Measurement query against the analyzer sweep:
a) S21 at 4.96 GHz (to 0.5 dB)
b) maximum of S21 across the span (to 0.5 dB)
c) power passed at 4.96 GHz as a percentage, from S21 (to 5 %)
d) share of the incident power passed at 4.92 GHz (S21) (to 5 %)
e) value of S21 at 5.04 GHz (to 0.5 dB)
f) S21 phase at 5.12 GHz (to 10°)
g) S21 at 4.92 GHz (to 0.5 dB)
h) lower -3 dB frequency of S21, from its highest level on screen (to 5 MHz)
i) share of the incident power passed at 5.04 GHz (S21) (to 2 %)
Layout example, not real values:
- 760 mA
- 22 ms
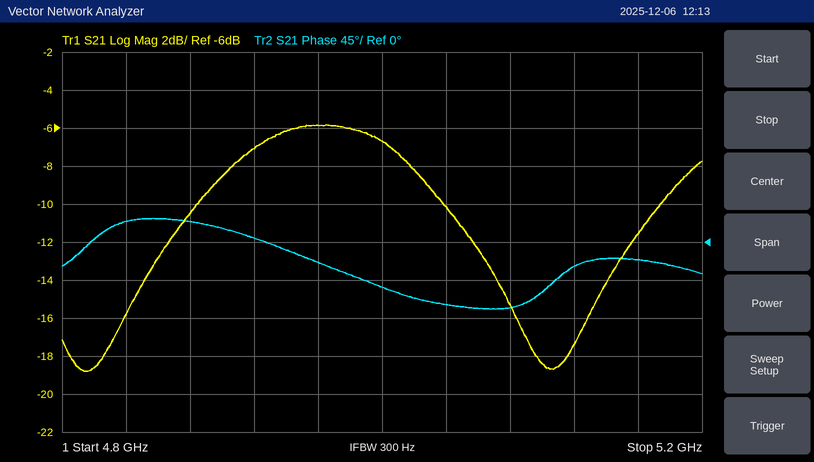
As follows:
- -6.0 dB
- -6.0 dB
- 25 %
- 20 %
- -10.0 dB
- -30°
- -7.0 dB
- 4.895 GHz
- 10 %
